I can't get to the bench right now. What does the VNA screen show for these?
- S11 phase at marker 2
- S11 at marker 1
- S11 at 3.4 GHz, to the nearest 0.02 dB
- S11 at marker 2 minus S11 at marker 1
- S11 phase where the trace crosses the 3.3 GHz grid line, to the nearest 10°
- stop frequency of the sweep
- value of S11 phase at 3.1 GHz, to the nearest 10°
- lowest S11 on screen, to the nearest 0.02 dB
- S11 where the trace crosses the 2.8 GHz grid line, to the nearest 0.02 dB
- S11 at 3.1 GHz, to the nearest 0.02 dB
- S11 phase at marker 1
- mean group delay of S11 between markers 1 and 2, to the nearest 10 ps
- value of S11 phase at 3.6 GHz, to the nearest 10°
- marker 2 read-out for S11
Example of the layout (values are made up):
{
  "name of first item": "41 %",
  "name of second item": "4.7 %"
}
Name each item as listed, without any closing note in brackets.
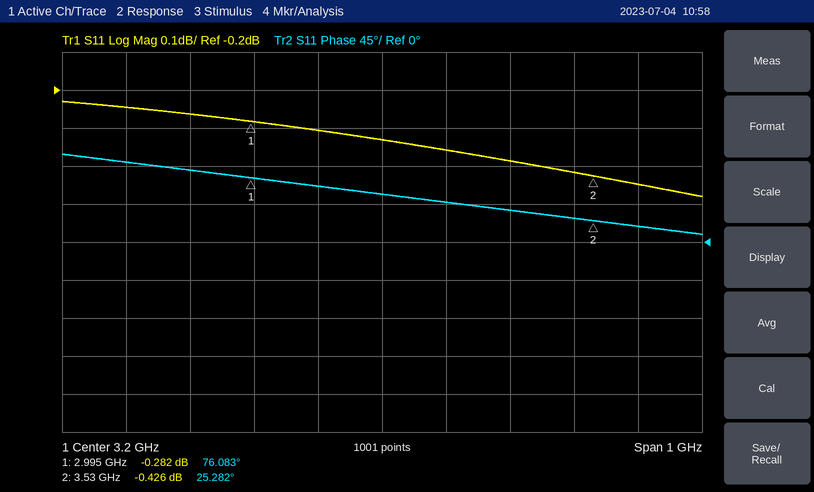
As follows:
{
  "S11 phase at marker 2": "25.282°",
  "S11 at marker 1": "-0.282 dB",
  "S11 at 3.4 GHz, to the nearest 0.02 dB": "-0.38 dB",
  "S11 at marker 2 minus S11 at marker 1": "-0.144 dB",
  "S11 phase where the trace crosses the 3.3 GHz grid line, to the nearest 10°": "50°",
  "stop frequency of the sweep": "3.7 GHz",
  "value of S11 phase at 3.1 GHz, to the nearest 10°": "70°",
  "lowest S11 on screen, to the nearest 0.02 dB": "-0.48 dB",
  "S11 where the trace crosses the 2.8 GHz grid line, to the nearest 0.02 dB": "-0.24 dB",
  "S11 at 3.1 GHz, to the nearest 0.02 dB": "-0.30 dB",
  "S11 phase at marker 1": "76.083°",
  "mean group delay of S11 between markers 1 and 2, to the nearest 10 ps": "260 ps",
  "value of S11 phase at 3.6 GHz, to the nearest 10°": "20°",
  "marker 2 read-out for S11": "-0.426 dB"
}
